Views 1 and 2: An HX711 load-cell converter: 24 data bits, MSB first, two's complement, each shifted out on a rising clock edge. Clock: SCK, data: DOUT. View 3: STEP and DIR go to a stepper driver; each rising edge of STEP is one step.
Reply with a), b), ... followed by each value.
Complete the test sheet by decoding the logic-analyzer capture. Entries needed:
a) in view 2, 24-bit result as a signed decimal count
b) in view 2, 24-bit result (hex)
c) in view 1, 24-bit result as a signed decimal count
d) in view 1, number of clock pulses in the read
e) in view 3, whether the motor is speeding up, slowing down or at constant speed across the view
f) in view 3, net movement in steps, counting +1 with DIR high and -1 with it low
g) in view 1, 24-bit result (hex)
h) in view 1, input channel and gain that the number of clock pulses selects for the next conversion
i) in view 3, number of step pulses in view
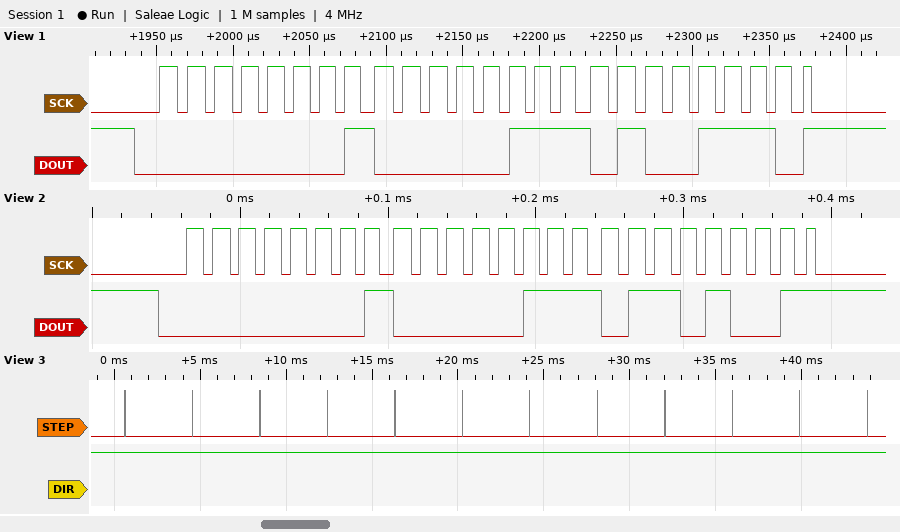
a) 67433
b) 0x010769
c) 67406
d) 25
e) constant speed
f) +12
g) 0x01074E
h) channel A, gain 128
i) 12
